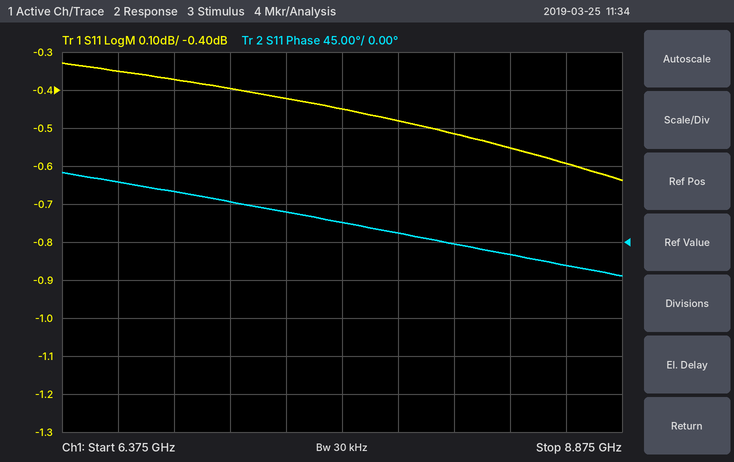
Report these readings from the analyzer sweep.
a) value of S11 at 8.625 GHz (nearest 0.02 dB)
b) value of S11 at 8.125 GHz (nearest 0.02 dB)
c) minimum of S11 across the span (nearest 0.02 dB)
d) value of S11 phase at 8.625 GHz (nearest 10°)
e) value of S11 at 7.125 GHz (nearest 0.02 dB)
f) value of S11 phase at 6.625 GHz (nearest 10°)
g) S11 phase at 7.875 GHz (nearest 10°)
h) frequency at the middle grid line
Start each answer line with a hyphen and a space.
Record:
- -0.60 dB
- -0.52 dB
- -0.64 dB
- -30°
- -0.40 dB
- 70°
- 10°
- 7.625 GHz
